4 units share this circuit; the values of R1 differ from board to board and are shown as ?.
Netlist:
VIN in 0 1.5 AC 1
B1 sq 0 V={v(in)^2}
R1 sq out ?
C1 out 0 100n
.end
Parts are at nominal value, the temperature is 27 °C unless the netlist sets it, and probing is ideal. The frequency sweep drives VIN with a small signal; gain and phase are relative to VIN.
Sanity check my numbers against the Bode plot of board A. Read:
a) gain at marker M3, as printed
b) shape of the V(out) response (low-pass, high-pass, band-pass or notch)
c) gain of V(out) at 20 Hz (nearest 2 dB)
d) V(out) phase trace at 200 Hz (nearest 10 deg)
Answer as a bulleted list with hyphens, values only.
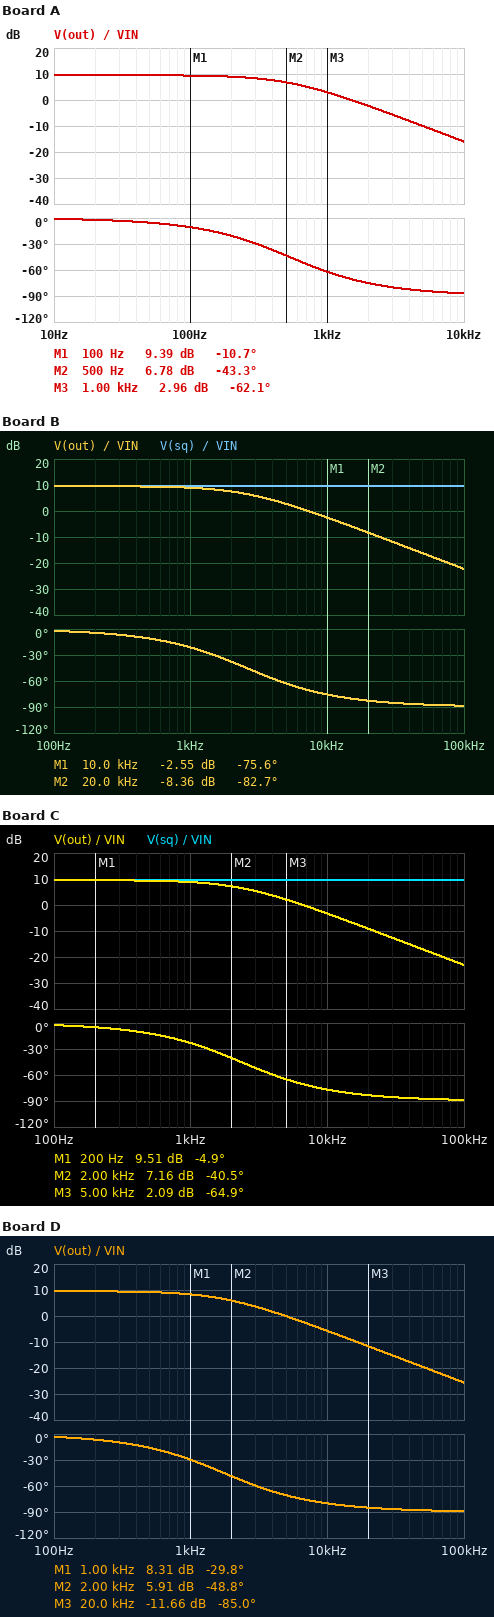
- 2.96 dB
- low-pass
- 10 dB
- -20 deg
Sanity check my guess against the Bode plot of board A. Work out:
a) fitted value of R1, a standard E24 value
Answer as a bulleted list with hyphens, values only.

- 3 kΩ
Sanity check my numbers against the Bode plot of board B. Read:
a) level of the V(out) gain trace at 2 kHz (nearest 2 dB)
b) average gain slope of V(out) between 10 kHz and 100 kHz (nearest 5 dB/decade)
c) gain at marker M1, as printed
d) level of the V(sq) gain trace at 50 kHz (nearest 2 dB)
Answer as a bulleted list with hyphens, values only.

- 8 dB
- -20 dB/decade
- -2.55 dB
- 10 dB
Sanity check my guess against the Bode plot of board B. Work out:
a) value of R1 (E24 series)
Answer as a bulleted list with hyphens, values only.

- 620 Ω
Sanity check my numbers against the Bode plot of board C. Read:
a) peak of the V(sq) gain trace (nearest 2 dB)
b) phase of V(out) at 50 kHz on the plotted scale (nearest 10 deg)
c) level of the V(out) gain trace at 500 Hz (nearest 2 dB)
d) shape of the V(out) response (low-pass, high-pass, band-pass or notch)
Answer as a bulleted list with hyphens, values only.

- 10 dB
- -90 deg
- 10 dB
- low-pass
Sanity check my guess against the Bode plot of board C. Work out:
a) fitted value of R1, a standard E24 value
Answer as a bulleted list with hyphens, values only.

- 680 Ω
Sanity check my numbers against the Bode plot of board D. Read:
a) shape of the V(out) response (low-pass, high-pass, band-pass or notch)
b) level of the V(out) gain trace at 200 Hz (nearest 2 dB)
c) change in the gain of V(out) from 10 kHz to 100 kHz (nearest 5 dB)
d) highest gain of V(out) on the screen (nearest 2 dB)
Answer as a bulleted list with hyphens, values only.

- low-pass
- 10 dB
- -20 dB
- 10 dB
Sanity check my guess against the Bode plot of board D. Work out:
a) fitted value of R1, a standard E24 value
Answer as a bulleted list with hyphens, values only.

- 910 Ω
